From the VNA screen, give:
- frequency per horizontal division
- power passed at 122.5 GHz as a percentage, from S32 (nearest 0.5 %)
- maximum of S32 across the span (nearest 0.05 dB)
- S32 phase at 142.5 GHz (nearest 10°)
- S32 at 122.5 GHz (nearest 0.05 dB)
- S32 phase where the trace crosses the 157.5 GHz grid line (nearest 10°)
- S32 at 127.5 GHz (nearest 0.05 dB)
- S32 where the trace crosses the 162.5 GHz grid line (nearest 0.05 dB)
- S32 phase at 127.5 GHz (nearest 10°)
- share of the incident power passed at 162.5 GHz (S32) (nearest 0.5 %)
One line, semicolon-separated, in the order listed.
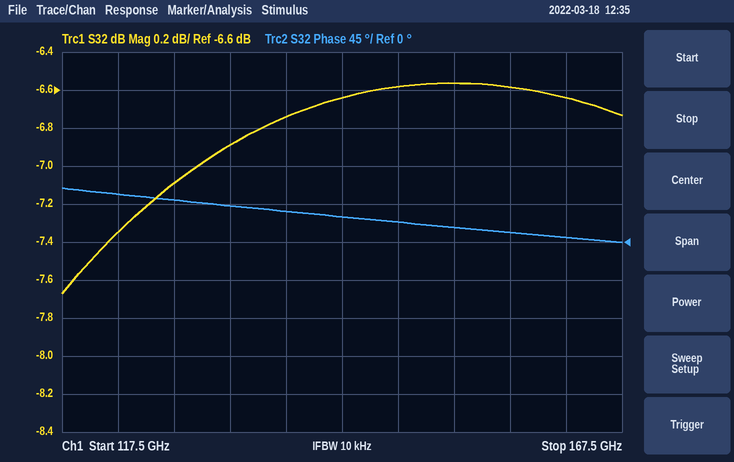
5 GHz; 18.5 %; -6.55 dB; 30°; -7.35 dB; 10°; -7.10 dB; -6.65 dB; 50°; 21.5 %
